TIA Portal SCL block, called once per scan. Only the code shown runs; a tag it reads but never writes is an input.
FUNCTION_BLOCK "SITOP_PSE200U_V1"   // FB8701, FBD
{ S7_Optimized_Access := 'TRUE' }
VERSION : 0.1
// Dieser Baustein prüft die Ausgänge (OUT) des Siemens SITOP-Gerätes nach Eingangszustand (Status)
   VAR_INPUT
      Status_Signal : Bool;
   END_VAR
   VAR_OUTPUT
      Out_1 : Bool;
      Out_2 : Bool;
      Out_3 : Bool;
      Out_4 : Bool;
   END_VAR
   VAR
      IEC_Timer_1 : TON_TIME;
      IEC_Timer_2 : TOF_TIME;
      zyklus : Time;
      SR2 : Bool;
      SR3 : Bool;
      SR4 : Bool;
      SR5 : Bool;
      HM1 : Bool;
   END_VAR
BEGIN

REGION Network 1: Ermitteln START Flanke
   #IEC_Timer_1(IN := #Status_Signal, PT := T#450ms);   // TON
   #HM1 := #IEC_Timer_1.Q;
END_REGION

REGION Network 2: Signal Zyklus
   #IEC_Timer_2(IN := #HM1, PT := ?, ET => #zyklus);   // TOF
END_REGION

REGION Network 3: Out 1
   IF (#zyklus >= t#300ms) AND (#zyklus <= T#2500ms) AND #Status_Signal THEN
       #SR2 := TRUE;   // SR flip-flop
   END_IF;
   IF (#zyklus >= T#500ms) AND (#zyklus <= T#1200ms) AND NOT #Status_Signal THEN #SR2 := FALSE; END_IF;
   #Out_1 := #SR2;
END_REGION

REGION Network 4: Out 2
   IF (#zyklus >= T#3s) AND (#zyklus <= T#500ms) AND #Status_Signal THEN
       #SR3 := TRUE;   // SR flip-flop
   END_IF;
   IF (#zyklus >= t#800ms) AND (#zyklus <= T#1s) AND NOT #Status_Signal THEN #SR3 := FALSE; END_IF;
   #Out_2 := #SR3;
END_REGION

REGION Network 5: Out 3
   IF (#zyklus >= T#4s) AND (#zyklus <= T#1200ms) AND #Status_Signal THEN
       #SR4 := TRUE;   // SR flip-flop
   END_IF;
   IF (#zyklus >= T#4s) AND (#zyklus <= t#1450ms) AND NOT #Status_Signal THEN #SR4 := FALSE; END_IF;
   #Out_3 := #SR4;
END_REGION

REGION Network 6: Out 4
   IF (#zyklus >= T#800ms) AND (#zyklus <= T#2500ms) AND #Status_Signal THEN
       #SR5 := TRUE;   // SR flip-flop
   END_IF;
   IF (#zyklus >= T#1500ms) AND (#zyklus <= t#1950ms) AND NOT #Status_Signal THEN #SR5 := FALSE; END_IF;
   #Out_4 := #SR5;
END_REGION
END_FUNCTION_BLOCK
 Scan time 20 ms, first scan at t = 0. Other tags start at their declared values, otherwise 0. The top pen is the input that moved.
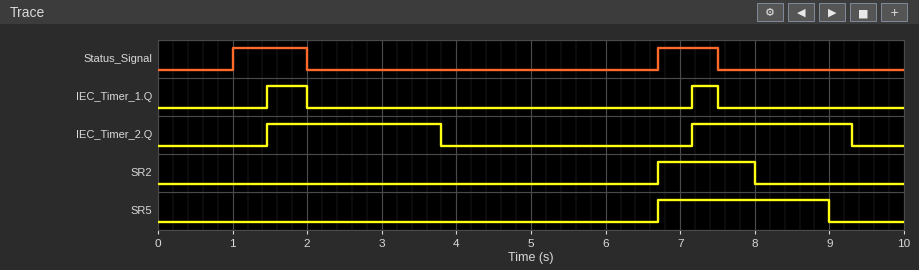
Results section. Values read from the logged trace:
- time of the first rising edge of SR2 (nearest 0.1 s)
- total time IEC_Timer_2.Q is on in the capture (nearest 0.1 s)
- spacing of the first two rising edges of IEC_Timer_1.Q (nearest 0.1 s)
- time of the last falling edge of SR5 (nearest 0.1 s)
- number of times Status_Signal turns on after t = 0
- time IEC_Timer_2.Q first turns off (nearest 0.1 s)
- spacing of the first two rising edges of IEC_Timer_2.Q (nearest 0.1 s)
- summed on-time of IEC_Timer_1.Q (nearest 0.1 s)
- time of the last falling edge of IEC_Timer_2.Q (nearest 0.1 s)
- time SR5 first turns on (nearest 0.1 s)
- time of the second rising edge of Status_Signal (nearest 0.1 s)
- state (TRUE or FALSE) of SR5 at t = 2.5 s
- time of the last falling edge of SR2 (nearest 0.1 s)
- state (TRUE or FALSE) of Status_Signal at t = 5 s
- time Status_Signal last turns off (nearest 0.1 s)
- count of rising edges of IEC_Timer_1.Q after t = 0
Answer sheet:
6.7 s
4.5 s
5.7 s
9.0 s
2
3.8 s
5.7 s
0.9 s
9.3 s
6.7 s
6.7 s
FALSE
8.0 s
FALSE
7.5 s
2
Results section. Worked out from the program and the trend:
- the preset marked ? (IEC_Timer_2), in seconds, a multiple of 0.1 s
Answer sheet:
1.8 s
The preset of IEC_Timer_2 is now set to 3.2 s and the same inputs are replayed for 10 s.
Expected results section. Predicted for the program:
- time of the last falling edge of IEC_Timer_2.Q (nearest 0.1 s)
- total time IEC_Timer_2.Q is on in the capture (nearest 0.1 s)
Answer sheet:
5.2 s
6.6 s
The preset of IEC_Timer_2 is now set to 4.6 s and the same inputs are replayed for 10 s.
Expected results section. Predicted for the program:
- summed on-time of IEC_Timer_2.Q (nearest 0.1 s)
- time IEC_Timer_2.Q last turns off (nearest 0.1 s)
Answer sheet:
8.0 s
6.6 s
